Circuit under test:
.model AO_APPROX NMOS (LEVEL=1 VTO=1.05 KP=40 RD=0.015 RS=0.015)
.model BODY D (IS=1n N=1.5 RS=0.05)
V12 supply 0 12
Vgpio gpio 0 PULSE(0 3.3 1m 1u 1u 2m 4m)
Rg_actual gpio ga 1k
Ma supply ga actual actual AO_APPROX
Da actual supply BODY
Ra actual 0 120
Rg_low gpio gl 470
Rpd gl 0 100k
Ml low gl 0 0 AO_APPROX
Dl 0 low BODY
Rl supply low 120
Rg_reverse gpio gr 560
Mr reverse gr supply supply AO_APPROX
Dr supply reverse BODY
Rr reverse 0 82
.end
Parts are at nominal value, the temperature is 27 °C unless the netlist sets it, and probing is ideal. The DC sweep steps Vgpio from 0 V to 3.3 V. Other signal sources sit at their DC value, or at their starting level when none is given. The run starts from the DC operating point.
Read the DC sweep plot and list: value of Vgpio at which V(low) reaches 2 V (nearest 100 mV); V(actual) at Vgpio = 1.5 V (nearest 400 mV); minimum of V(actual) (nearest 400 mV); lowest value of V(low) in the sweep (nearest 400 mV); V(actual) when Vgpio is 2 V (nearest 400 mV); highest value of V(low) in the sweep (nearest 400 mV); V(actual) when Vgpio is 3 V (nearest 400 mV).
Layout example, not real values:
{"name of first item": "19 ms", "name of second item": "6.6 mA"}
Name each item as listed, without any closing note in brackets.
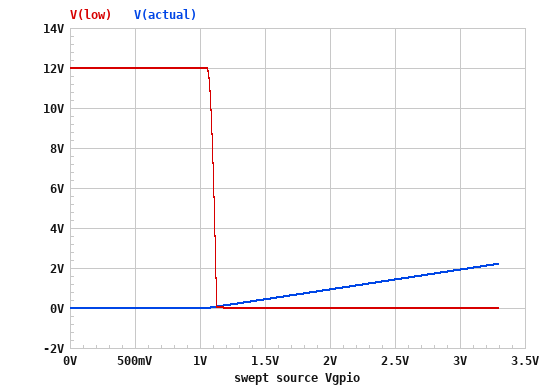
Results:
{"value of Vgpio at which V(low) reaches 2 V": "1.1 V", "V(actual) at Vgpio = 1.5 V": "400 mV", "minimum of V(actual)": "0 V", "lowest value of V(low) in the sweep": "0 V", "V(actual) when Vgpio is 2 V": "800 mV", "highest value of V(low) in the sweep": "12.0 V", "V(actual) when Vgpio is 3 V": "2.0 V"}
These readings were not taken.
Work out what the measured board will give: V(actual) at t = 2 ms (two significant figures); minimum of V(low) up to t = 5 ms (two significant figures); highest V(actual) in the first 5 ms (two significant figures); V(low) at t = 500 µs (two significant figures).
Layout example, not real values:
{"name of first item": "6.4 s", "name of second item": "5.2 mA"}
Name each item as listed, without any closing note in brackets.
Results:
{"V(actual) at t = 2 ms": "2.2 V", "minimum of V(low) up to t = 5 ms": "4.1 mV", "highest V(actual) in the first 5 ms": "2.2 V", "V(low) at t = 500 µs": "12 V"}
